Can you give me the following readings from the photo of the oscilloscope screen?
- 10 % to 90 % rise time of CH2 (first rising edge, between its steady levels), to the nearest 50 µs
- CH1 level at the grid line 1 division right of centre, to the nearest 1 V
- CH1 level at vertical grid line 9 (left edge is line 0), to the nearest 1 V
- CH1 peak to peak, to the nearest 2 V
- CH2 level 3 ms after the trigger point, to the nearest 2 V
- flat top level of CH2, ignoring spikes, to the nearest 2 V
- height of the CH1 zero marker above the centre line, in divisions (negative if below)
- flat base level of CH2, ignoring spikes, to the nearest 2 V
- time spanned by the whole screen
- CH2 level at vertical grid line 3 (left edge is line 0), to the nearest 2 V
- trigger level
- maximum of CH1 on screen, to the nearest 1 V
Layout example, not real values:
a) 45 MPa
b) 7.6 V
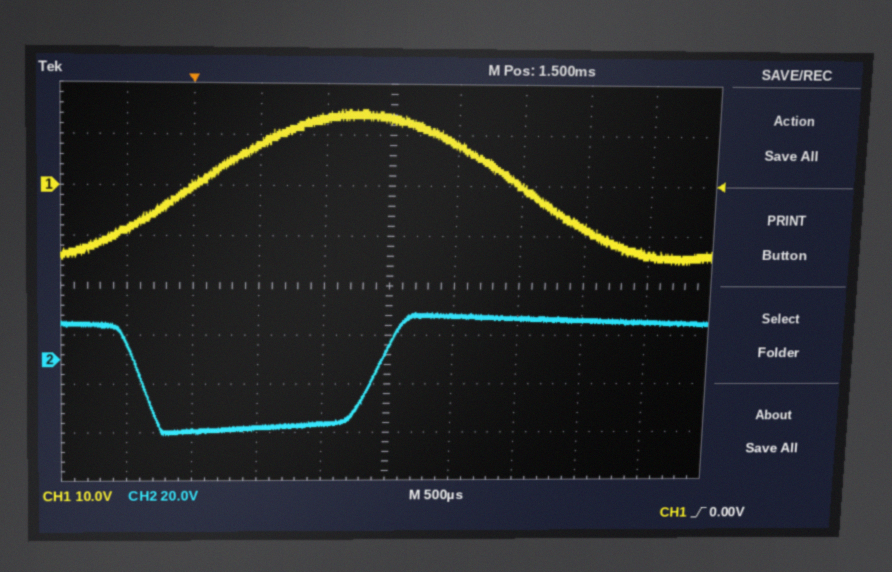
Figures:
a) 350 µs
b) 8 V
c) -14 V
d) 30 V
e) 16 V
f) 16 V
g) +2.0 div
h) -28 V
i) 5 ms
j) -28 V
k) 0.00 V
l) 15 V
